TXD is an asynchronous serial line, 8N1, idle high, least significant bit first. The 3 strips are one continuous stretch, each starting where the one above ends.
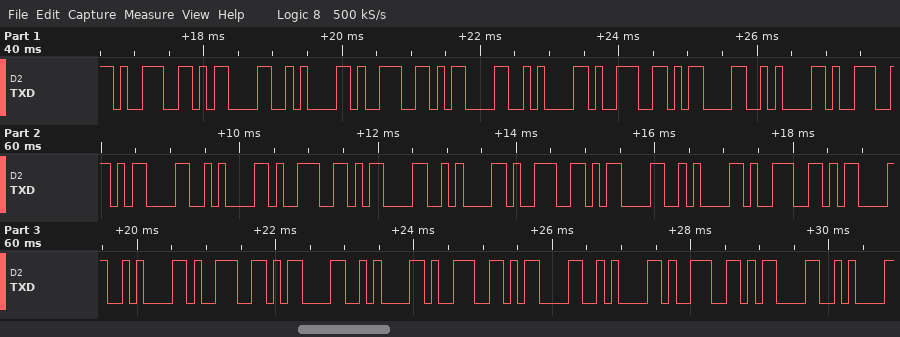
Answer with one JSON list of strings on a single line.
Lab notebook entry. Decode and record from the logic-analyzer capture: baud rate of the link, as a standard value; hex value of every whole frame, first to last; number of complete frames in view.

["9600 baud", "39 0D 0A 39 0D 0A 39 0D 0A 39 0D 0A 39 0D 0A 39 0D 0A 39 0D 0A 39 0D 0A 39 0D 0A 39 0D 0A", "30"]
